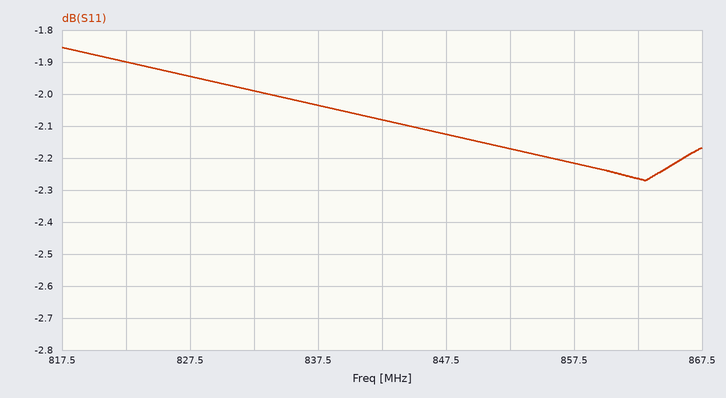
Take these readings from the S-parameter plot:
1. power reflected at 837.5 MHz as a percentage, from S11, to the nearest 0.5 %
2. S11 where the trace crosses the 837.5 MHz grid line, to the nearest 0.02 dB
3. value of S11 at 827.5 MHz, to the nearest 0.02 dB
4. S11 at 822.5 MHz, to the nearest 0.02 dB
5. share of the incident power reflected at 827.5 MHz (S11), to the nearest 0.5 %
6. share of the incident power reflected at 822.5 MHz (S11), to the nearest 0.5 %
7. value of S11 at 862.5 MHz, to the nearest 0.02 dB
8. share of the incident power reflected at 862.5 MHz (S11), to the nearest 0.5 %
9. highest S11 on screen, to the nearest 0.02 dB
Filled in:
62.5 %
-2.04 dB
-1.94 dB
-1.90 dB
64.0 %
64.5 %
-2.26 dB
59.5 %
-1.86 dB
